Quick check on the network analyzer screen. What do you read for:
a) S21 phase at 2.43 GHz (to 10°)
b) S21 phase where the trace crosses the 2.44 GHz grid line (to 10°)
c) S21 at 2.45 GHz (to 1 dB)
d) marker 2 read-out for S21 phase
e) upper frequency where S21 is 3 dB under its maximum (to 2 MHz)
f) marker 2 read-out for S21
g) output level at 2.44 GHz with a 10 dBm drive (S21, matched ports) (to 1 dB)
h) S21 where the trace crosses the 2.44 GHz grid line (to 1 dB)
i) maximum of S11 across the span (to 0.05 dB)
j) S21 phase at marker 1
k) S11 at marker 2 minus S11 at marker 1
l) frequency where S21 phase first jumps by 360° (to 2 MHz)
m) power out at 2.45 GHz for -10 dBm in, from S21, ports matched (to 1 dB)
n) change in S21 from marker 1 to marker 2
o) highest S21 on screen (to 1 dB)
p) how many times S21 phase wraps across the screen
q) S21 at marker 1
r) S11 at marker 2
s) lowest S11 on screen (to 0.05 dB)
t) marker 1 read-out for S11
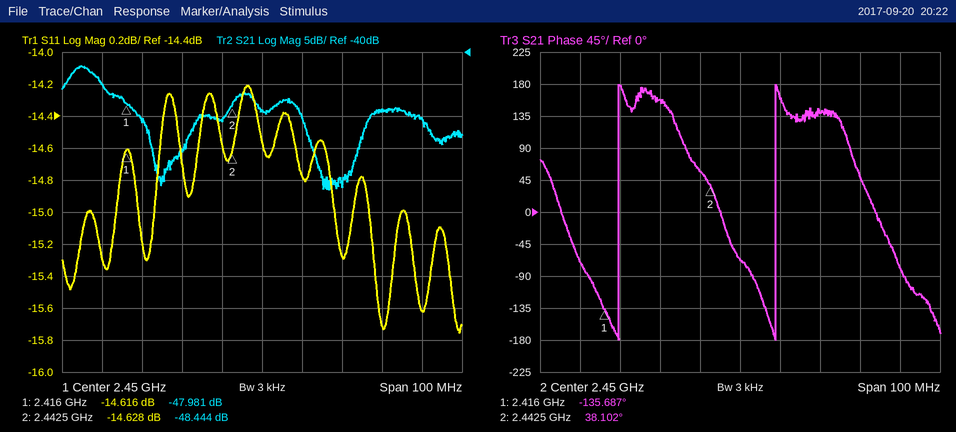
160°
60°
-49 dB
38.102°
2.410 GHz
-48.444 dB
-41 dBm
-51 dB
-14.20 dB
-135.687°
-0.012 dB
2.420 GHz
-59 dBm
-0.463 dB
-42 dB
2
-47.981 dB
-14.628 dB
-15.75 dB
-14.616 dB
